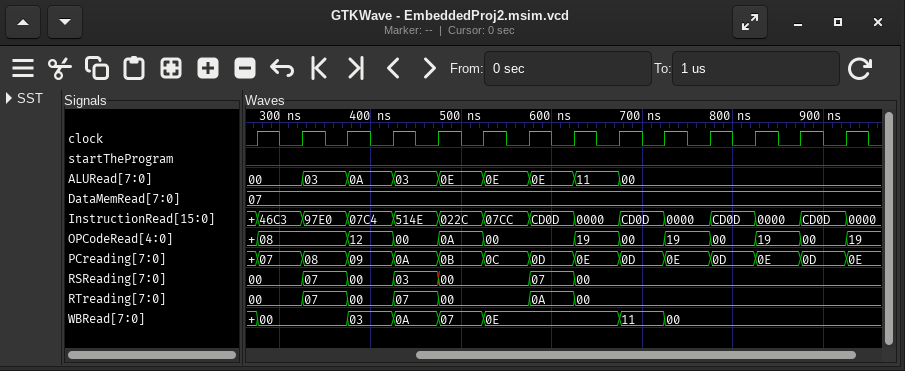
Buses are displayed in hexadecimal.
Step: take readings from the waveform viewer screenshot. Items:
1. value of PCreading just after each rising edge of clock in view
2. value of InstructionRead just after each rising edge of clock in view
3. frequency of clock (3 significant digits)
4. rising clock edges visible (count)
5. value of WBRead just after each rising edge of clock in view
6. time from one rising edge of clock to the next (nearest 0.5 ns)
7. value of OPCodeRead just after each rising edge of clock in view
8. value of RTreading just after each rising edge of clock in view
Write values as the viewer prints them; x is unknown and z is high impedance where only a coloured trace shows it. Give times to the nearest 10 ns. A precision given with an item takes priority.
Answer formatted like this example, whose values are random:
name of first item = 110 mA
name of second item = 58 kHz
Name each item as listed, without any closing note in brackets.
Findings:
value of PCreading just after each rising edge of clock in view = 07, 08, 09, 0A, 0B, 0C, 0D, 0E, 0D, 0E, 0D, 0E, 0D, 0E
value of InstructionRead just after each rising edge of clock in view = 46C3, 97E0, 07C4, 514E, 022C, 07CC, CD0D, 0000, CD0D, 0000, CD0D, 0000, CD0D, 0000
frequency of clock = 20.0 MHz
rising clock edges visible = 14
value of WBRead just after each rising edge of clock in view = 00, 00, 03, 0A, 07, 0E, 0E, 0E, 11, 00, 00, 00, 00, 00
time from one rising edge of clock to the next = 50 ns
value of OPCodeRead just after each rising edge of clock in view = 08, 08, 12, 00, 0A, 00, 00, 19, 00, 19, 00, 19, 00, 19
value of RTreading just after each rising edge of clock in view = 00, 07, 00, 07, 00, 00, 0A, 00, 00, 00, 00, 00, 00, 00
